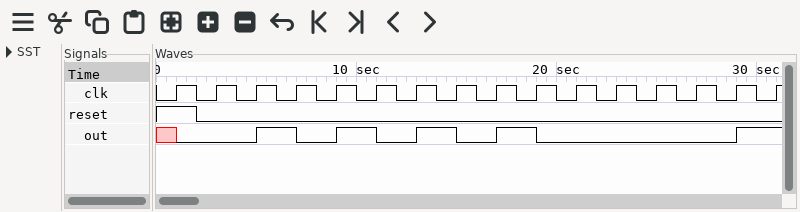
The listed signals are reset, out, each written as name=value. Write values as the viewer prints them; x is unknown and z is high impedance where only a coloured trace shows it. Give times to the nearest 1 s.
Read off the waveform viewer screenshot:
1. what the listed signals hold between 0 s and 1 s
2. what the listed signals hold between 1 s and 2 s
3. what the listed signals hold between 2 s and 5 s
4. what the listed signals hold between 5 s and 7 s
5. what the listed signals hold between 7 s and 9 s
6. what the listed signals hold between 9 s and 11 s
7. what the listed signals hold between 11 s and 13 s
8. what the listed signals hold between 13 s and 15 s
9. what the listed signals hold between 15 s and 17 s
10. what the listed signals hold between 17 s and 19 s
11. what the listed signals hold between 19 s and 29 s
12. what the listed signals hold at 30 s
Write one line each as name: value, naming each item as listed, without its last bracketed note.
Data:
what the listed signals hold between 0 s and 1 s: reset=1, out=x
what the listed signals hold between 1 s and 2 s: reset=1, out=0
what the listed signals hold between 2 s and 5 s: reset=0, out=0
what the listed signals hold between 5 s and 7 s: reset=0, out=1
what the listed signals hold between 7 s and 9 s: reset=0, out=0
what the listed signals hold between 9 s and 11 s: reset=0, out=1
what the listed signals hold between 11 s and 13 s: reset=0, out=0
what the listed signals hold between 13 s and 15 s: reset=0, out=1
what the listed signals hold between 15 s and 17 s: reset=0, out=0
what the listed signals hold between 17 s and 19 s: reset=0, out=1
what the listed signals hold between 19 s and 29 s: reset=0, out=0
what the listed signals hold at 30 s: reset=0, out=1
